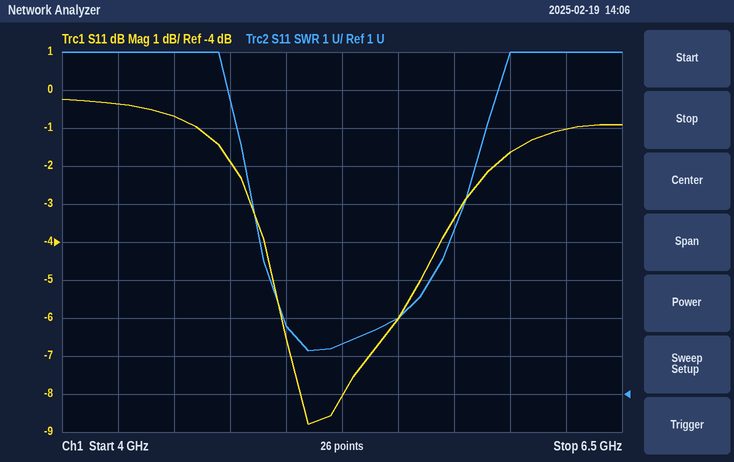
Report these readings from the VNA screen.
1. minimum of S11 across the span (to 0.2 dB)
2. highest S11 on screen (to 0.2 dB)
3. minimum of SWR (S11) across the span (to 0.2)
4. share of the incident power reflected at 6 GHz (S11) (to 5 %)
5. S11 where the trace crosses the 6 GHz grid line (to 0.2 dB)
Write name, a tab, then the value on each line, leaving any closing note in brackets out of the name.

minimum of S11 across the span	-8.8 dB
highest S11 on screen	-0.2 dB
minimum of SWR (S11) across the span	2.2
share of the incident power reflected at 6 GHz (S11)	70 %
S11 where the trace crosses the 6 GHz grid line	-1.6 dB
